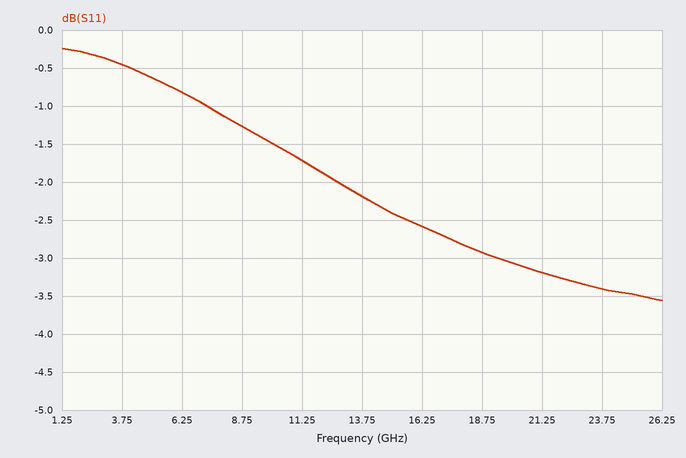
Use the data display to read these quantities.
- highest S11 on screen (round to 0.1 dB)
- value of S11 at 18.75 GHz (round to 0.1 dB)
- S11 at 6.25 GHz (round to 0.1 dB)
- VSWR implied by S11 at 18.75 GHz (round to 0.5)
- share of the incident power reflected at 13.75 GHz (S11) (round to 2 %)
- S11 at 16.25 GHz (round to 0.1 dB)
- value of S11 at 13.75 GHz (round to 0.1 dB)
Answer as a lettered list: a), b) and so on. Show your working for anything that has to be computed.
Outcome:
a) -0.2 dB
b) -2.9 dB
c) -0.8 dB
d) |Γ| = 10^(-2.9/20) = 0.7161; VSWR = (1 + 0.7161)/(1 − 0.7161) ≈ 6.0
e) 10^(-2.2/10) ≈ 60 %
f) -2.6 dB
g) -2.2 dB
